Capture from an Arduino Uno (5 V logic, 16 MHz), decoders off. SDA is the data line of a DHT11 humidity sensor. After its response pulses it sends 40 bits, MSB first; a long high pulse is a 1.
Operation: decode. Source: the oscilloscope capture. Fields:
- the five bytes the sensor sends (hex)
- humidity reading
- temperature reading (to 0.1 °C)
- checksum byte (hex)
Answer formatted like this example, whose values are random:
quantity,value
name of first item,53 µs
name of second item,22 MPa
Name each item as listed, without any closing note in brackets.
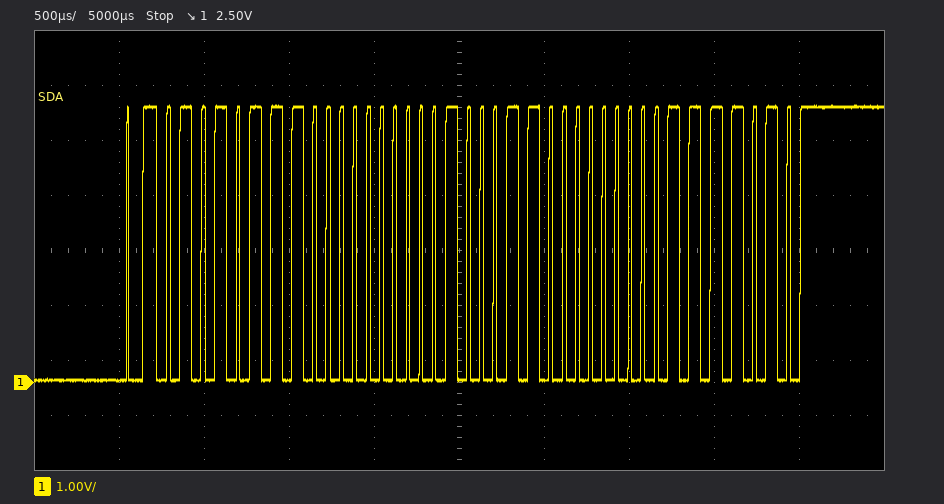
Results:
quantity,value
the five bytes the sensor sends,57 00 23 00 7A
humidity reading,87 %
temperature reading,35.0 °C
checksum byte,0x7A
